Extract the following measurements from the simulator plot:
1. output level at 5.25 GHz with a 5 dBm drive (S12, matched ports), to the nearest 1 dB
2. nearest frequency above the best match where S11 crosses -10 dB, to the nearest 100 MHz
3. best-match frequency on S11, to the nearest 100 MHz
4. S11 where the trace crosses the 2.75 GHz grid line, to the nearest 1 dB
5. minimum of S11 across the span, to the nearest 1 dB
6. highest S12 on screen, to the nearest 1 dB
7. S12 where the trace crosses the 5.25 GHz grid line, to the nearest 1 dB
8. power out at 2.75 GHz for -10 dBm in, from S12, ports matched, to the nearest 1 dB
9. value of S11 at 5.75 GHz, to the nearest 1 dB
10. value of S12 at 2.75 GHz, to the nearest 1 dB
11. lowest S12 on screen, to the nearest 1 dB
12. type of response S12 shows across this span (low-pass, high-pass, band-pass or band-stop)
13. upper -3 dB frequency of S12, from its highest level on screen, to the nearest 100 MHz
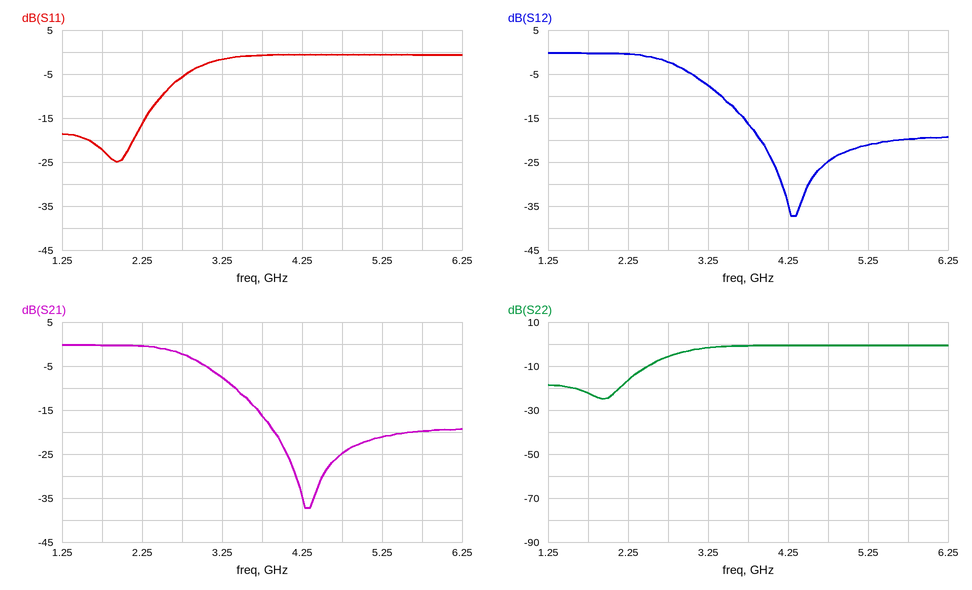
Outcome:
-16 dBm
2.5 GHz
1.9 GHz
-6 dB
-25 dB
0 dB
-21 dB
-12 dBm
-1 dB
-2 dB
-37 dB
low-pass
2.9 GHz
